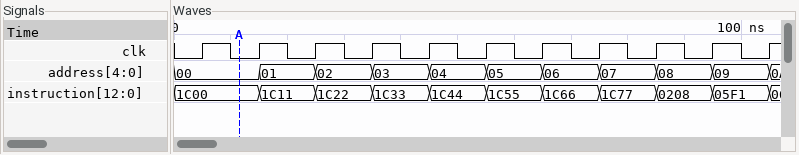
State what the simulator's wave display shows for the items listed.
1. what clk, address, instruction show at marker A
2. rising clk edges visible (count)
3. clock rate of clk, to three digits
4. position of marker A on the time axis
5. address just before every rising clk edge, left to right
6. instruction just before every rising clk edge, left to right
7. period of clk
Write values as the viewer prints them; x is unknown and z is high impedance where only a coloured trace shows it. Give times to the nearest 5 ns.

clk=0, address=00, instruction=1C00
11
100 MHz
10 ns
00, 00, 01, 02, 03, 04, 05, 06, 07, 08, 09
1C00, 1C00, 1C11, 1C22, 1C33, 1C44, 1C55, 1C66, 1C77, 0208, 05F1
10 ns
